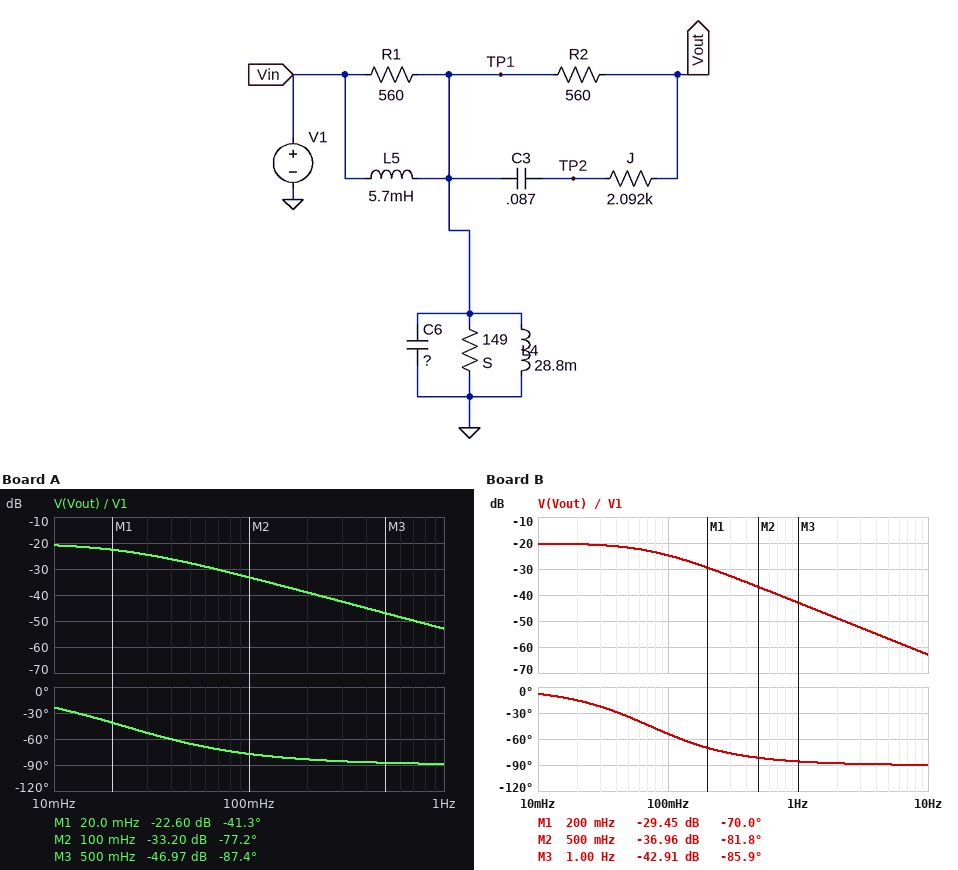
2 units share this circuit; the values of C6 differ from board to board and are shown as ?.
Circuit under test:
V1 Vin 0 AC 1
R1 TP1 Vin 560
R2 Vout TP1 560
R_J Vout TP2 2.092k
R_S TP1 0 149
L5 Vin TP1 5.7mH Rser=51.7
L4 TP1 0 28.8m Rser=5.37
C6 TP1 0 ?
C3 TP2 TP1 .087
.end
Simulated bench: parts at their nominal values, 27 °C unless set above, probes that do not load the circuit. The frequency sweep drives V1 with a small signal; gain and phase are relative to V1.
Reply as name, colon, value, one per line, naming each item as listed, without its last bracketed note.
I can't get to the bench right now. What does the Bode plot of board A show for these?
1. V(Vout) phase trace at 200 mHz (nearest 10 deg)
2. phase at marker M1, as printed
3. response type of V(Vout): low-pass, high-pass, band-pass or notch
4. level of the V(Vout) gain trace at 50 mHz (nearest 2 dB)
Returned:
V(Vout) phase trace at 200 mHz: -80 deg
phase at marker M1, as printed: -41.3 deg
response type of V(Vout): low-pass, high-pass, band-pass or notch: low-pass
level of the V(Vout) gain trace at 50 mHz: -28 dB
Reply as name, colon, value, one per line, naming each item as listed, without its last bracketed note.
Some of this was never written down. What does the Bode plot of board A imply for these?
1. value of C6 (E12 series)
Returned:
value of C6: 1.5 F
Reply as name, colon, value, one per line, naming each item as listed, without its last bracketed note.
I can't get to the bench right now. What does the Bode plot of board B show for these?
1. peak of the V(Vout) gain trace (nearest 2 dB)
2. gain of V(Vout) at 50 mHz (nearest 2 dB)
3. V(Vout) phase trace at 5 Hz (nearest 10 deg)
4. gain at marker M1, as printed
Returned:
peak of the V(Vout) gain trace: -20 dB
gain of V(Vout) at 50 mHz: -22 dB
V(Vout) phase trace at 5 Hz: -90 deg
gain at marker M1, as printed: -29.45 dB
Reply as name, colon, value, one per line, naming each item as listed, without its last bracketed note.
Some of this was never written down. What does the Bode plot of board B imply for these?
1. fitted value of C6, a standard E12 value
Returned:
fitted value of C6, a standard E12 value: 470 mF
